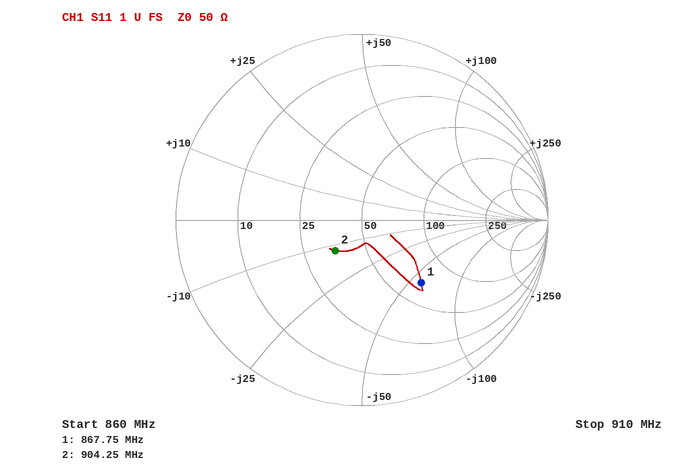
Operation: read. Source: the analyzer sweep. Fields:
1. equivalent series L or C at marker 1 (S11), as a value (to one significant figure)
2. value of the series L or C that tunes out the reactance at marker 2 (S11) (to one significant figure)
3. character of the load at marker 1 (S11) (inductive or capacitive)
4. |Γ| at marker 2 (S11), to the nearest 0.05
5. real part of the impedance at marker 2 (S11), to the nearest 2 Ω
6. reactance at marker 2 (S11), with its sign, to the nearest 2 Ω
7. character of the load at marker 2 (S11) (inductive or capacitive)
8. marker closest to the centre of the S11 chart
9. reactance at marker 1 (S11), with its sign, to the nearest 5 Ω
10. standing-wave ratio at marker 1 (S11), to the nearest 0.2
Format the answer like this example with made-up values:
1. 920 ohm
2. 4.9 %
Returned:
1. 3 pF
2. 2 nH
3. capacitive
4. 0.20
5. 36 Ω
6. -12 Ω
7. capacitive
8. marker 2
9. -60 Ω
10. 2.8
